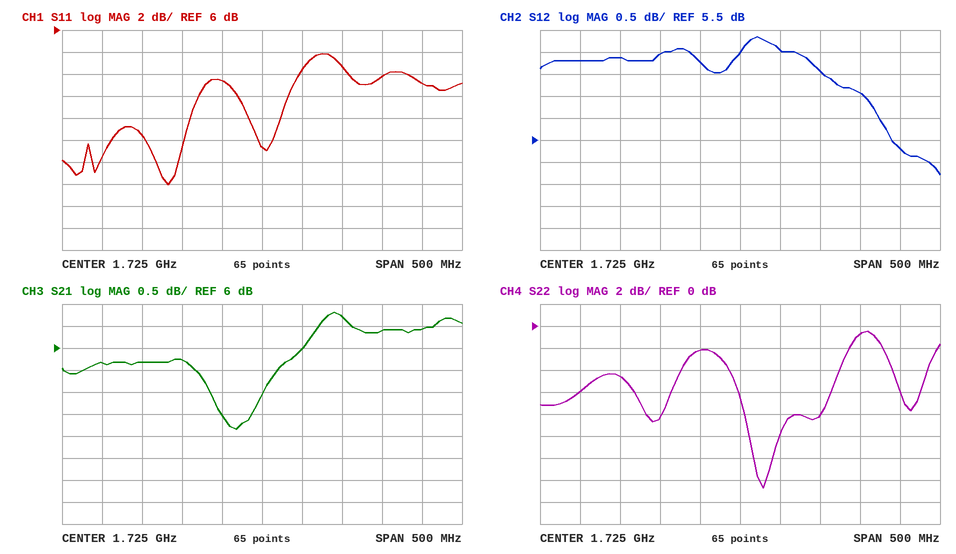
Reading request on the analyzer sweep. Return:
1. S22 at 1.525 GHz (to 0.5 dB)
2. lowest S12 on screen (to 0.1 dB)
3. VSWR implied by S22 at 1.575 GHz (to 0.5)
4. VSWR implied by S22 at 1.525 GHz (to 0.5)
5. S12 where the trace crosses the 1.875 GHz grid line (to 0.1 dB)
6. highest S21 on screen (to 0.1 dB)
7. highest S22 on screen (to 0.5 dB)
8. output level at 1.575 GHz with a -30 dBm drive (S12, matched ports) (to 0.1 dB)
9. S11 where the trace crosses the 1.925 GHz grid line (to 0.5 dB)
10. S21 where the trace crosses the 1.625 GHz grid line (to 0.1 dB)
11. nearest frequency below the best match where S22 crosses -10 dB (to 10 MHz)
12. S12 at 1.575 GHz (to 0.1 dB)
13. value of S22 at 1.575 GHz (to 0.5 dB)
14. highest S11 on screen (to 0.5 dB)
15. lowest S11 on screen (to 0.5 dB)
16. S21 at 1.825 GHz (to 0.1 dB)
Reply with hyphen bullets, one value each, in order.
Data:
- -6.0 dB
- 4.7 dB
- 4.0
- 3.0
- 6.6 dB
- 6.8 dB
- -0.5 dB
- -22.6 dBm
- 1.0 dB
- 5.7 dB
- 1.74 GHz
- 7.4 dB
- -4.5 dB
- 4.0 dB
- -8.0 dB
- 6.7 dB
